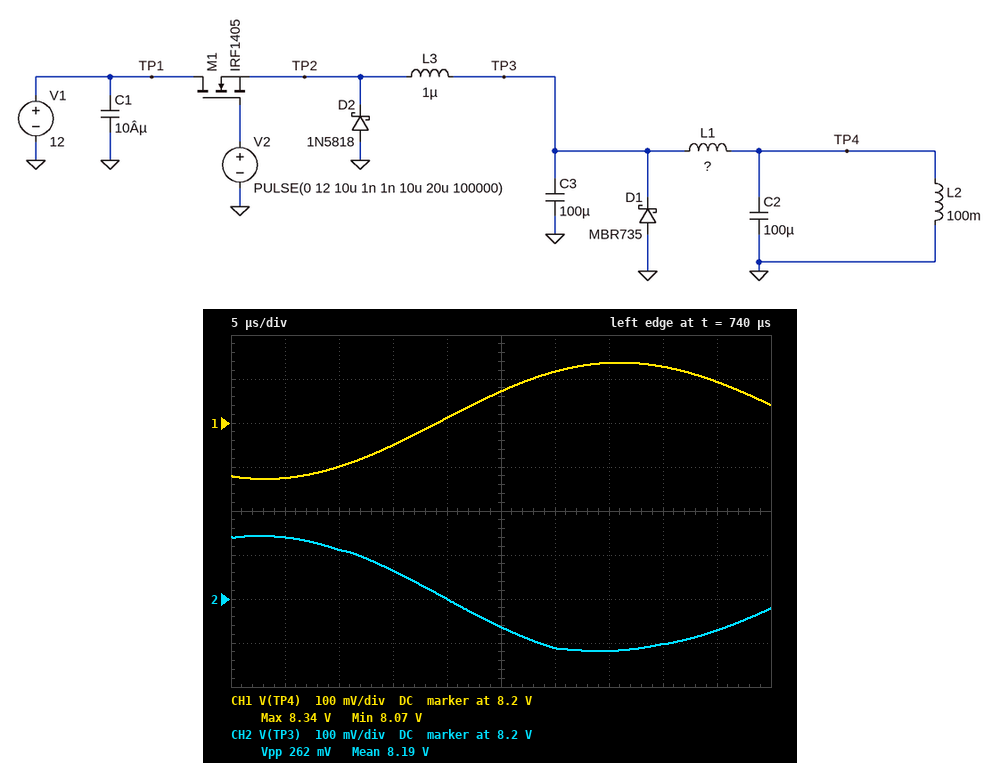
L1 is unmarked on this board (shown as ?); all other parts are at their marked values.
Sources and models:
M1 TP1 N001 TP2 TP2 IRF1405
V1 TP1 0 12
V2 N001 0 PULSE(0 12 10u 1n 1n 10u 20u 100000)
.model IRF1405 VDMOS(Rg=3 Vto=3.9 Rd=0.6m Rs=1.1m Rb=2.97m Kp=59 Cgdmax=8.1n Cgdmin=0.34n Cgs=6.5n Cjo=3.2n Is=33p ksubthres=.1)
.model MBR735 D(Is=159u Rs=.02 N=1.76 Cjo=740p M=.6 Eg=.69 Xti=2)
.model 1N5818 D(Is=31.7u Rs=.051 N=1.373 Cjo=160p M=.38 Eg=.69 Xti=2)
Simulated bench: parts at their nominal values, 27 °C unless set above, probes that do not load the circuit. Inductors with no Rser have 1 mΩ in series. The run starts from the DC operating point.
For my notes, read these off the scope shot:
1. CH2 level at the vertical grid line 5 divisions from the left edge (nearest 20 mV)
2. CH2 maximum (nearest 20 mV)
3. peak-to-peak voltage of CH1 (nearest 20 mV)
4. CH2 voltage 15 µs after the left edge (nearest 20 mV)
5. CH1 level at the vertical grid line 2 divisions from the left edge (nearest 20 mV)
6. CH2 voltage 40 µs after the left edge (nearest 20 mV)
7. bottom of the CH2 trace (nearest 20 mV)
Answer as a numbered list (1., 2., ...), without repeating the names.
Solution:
1. 8.14 V
2. 8.34 V
3. 260 mV
4. 8.26 V
5. 8.10 V
6. 8.10 V
7. 8.08 V
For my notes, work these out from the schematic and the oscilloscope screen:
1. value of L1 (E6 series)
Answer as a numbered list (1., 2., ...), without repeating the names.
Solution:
1. 2.2 µH
